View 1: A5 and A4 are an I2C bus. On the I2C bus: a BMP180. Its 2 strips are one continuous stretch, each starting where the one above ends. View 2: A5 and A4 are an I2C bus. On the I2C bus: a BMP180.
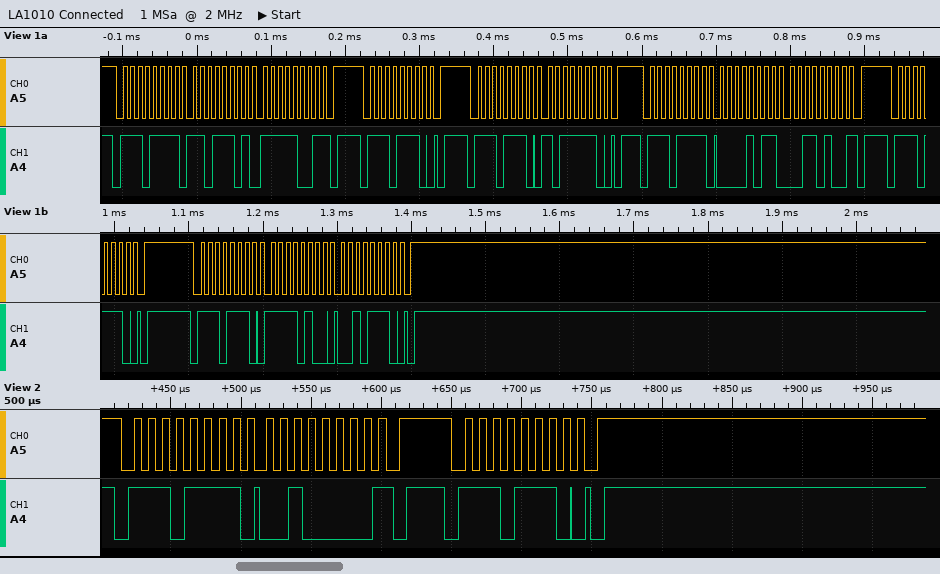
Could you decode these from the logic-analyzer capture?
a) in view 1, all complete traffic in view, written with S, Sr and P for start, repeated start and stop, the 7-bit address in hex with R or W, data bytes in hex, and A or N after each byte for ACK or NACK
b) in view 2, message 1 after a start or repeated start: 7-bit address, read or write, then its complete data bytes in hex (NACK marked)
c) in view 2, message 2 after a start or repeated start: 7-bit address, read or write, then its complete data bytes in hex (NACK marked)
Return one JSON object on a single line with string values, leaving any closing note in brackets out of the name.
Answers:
{"in view 1, all complete traffic in view, written with S, Sr and P for start, repeated start and stop, the 7-bit address in hex with R or W, data bytes in hex, and A or N after each byte for ACK or NACK": "S 77R A DD A F9 N P S 77W A P S 77W A BE A P S 77R A 0B A 34 N P S 77W A P S 77W A F4 A 2E A P", "in view 2, message 1 after a start or repeated start: 7-bit address, read or write, then its complete data bytes in hex": "0x77 read: 20 NACK", "in view 2, message 2 after a start or repeated start: 7-bit address, read or write, then its complete data bytes in hex": "0x77 write"}
